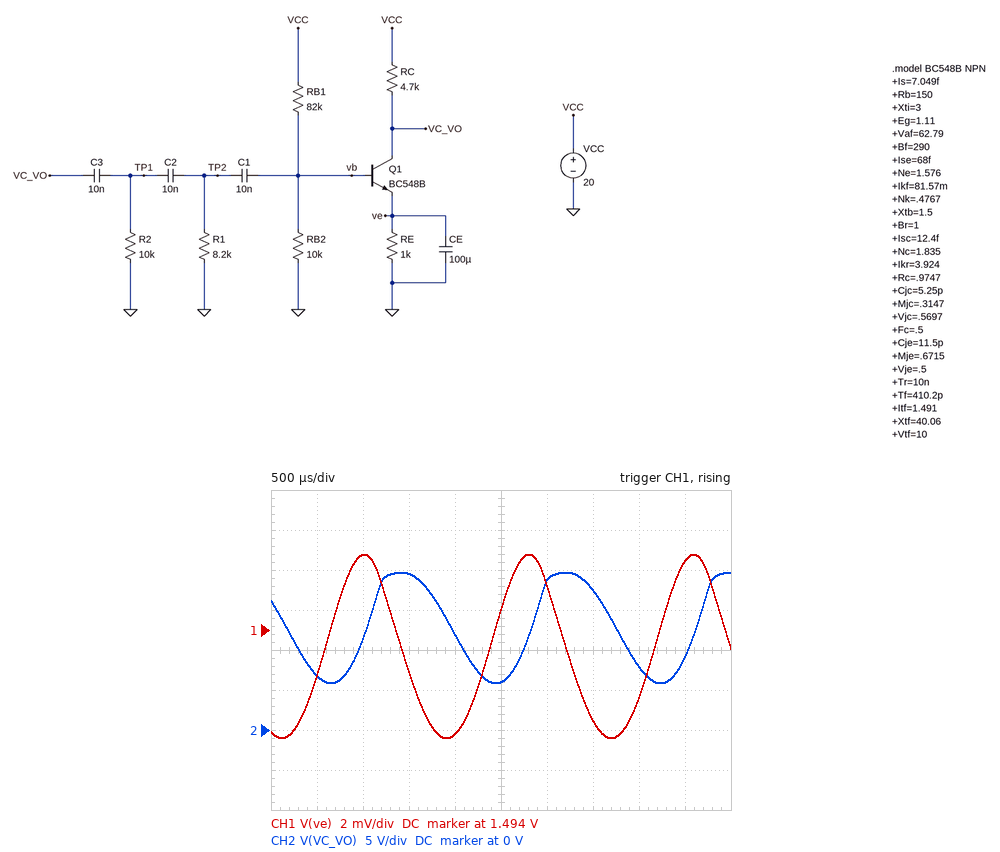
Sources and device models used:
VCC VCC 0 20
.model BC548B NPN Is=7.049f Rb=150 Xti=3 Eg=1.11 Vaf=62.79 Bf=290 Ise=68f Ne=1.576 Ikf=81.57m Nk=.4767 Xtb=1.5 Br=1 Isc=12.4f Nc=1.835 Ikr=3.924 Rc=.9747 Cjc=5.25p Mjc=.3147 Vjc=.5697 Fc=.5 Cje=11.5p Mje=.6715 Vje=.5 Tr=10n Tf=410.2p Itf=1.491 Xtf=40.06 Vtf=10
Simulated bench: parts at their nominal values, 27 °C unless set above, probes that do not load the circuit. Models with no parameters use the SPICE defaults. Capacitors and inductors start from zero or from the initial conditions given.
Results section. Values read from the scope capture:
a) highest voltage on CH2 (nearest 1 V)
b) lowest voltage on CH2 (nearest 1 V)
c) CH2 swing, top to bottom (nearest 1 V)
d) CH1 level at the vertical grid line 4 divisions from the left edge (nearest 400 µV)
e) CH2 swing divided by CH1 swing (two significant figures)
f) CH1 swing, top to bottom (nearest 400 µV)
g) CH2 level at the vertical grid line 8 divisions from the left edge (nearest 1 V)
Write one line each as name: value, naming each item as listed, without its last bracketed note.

highest voltage on CH2: 20 V
lowest voltage on CH2: 6 V
CH2 swing, top to bottom: 14 V
CH1 level at the vertical grid line 4 divisions from the left edge: 1.4888 V
CH2 swing divided by CH1 swing: 1500
CH1 swing, top to bottom: 9.2 mV
CH2 level at the vertical grid line 8 divisions from the left edge: 8 V
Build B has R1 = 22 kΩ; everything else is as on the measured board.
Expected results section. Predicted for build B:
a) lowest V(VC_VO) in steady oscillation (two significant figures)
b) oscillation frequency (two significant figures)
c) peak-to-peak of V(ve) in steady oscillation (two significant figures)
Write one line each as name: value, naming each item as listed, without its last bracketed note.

lowest V(VC_VO) in steady oscillation: 6.1 V
oscillation frequency: 410 Hz
peak-to-peak of V(ve) in steady oscillation: 12 mV
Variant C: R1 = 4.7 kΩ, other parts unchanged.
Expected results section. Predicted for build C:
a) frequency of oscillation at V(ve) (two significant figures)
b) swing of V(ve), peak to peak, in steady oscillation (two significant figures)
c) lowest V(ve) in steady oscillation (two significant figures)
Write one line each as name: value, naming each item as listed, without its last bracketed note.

frequency of oscillation at V(ve): 670 Hz
swing of V(ve), peak to peak, in steady oscillation: 7.7 mV
lowest V(ve) in steady oscillation: 1.5 V
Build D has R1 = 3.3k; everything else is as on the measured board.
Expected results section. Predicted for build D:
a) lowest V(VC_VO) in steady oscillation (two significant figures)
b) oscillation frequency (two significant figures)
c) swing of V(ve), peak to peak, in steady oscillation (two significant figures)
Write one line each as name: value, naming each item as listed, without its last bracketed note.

lowest V(VC_VO) in steady oscillation: 6.0 V
oscillation frequency: 750 Hz
swing of V(ve), peak to peak, in steady oscillation: 6.8 mV
